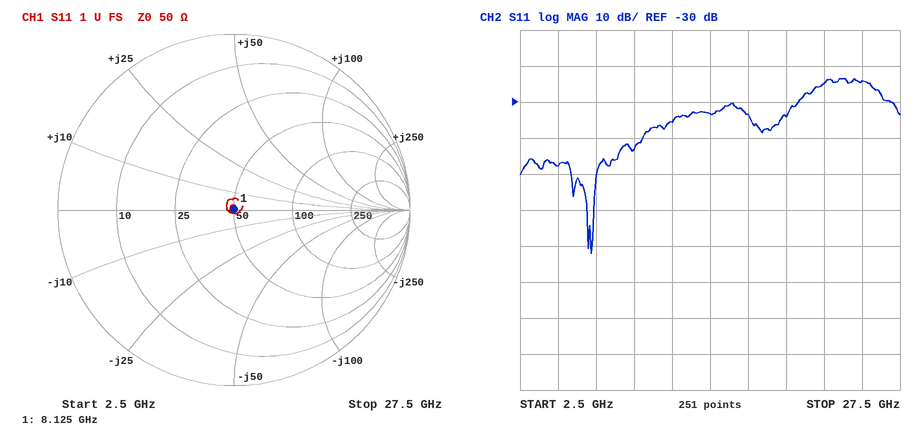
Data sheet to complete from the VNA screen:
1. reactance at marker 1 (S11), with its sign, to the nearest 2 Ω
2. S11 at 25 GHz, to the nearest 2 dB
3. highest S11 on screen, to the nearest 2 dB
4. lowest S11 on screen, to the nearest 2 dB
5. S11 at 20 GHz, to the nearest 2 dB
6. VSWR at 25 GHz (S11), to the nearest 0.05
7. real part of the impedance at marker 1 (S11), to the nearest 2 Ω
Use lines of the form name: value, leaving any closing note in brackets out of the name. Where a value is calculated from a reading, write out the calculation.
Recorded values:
reactance at marker 1 (S11), with its sign, to the nearest 2 Ω: 0 Ω
S11 at 25 GHz, to the nearest 2 dB: -24 dB
highest S11 on screen, to the nearest 2 dB: -24 dB
lowest S11 on screen, to the nearest 2 dB: -72 dB
S11 at 20 GHz, to the nearest 2 dB: -34 dB
VSWR at 25 GHz (S11), to the nearest 0.05: |Γ| = 10^(-24/20) = 0.0631; VSWR = (1 + 0.0631)/(1 − 0.0631) ≈ 1.13, so 1.15 to the nearest 0.05
real part of the impedance at marker 1 (S11), to the nearest 2 Ω: 50 Ω
